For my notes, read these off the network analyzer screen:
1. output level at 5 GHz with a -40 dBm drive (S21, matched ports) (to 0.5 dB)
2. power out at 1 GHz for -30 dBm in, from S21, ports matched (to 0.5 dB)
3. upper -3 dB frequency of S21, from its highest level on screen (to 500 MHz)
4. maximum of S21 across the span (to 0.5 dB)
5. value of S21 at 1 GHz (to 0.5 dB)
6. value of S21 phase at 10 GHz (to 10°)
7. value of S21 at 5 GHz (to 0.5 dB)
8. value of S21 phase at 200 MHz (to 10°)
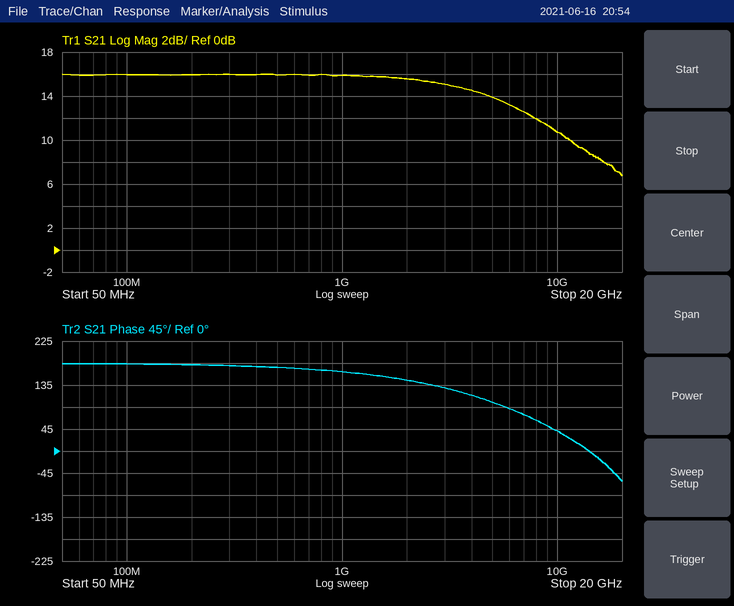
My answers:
-26.0 dBm
-14.0 dBm
6.5 GHz
16.0 dB
16.0 dB
40°
14.0 dB
180°
